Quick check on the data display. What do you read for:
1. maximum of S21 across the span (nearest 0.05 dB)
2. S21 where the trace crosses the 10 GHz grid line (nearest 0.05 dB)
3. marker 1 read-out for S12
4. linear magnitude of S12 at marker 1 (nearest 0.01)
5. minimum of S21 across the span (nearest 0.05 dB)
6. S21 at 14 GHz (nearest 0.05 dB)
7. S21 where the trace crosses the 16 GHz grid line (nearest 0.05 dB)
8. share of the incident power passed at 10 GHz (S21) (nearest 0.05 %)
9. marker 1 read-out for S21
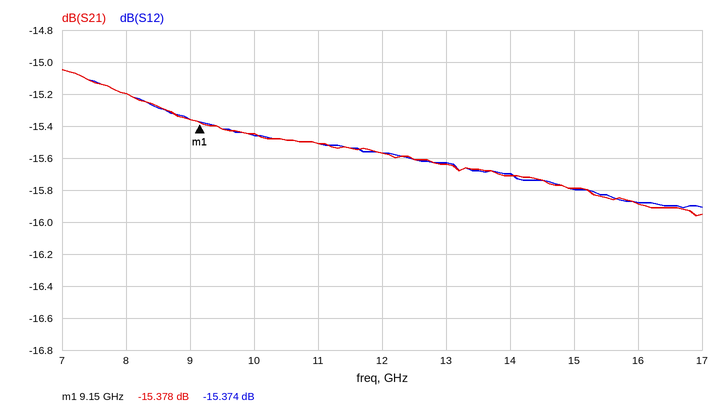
-15.05 dB
-15.45 dB
-15.374 dB
0.17
-15.95 dB
-15.70 dB
-15.90 dB
2.85 %
-15.378 dB
